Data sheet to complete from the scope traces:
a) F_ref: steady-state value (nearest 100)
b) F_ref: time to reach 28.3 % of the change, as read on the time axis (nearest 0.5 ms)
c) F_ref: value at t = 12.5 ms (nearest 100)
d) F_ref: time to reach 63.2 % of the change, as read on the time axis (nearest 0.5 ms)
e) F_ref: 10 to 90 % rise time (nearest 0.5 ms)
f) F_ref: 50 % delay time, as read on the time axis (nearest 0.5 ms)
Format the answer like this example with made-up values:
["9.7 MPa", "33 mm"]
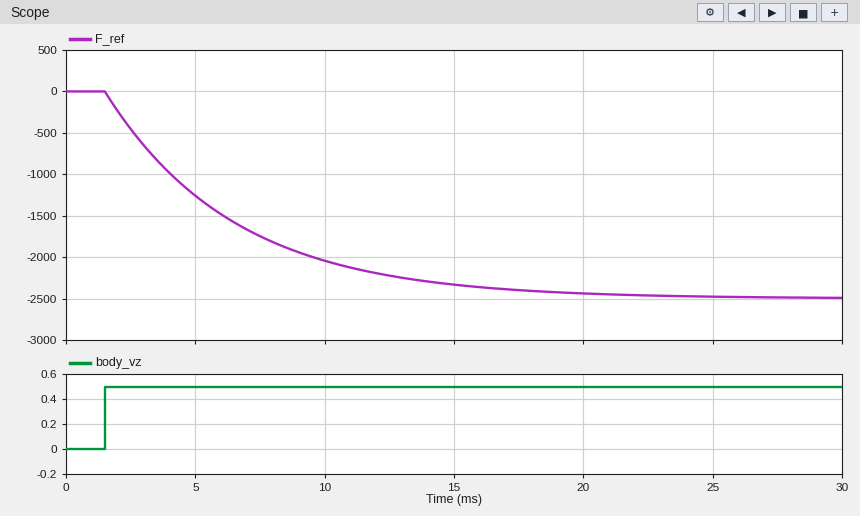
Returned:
["-2500", "3.0 ms", "-2200", "6.5 ms", "11.0 ms", "5.0 ms"]
